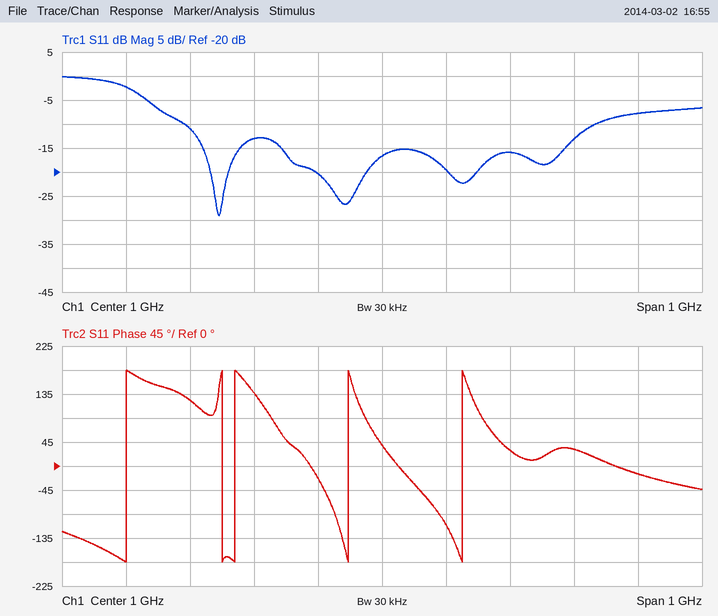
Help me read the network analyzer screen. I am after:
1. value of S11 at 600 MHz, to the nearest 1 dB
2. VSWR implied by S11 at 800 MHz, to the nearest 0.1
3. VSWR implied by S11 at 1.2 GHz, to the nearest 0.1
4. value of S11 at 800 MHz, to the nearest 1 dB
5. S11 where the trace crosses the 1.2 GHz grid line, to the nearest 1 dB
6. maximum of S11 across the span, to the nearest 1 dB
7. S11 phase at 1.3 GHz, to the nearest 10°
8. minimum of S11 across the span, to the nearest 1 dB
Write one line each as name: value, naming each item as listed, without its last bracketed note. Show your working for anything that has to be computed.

value of S11 at 600 MHz, to the nearest 1 dB: -2 dB
VSWR implied by S11 at 800 MHz, to the nearest 0.1: |Γ| = 10^(-13/20) = 0.2239; VSWR = (1 + 0.2239)/(1 − 0.2239) ≈ 1.6
VSWR implied by S11 at 1.2 GHz, to the nearest 0.1: |Γ| = 10^(-16/20) = 0.1585; VSWR = (1 + 0.1585)/(1 − 0.1585) ≈ 1.4
value of S11 at 800 MHz, to the nearest 1 dB: -13 dB
S11 where the trace crosses the 1.2 GHz grid line, to the nearest 1 dB: -16 dB
maximum of S11 across the span, to the nearest 1 dB: 0 dB
S11 phase at 1.3 GHz, to the nearest 10°: 30°
minimum of S11 across the span, to the nearest 1 dB: -29 dB
